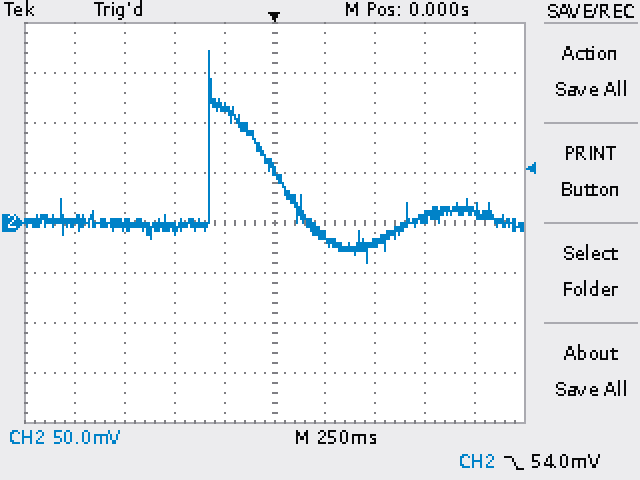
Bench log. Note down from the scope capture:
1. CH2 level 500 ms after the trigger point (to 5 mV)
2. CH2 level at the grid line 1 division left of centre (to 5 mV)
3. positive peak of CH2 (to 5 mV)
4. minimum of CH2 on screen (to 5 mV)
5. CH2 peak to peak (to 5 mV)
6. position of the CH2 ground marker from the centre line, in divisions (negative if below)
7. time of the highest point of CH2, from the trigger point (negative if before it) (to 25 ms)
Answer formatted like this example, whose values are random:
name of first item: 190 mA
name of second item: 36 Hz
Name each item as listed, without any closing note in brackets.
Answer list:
CH2 level 500 ms after the trigger point: -20 mV
CH2 level at the grid line 1 division left of centre: 115 mV
positive peak of CH2: 170 mV
minimum of CH2 on screen: -40 mV
CH2 peak to peak: 210 mV
position of the CH2 ground marker from the centre line, in divisions: 0.0 div
time of the highest point of CH2, from the trigger point (negative if before it): -325 ms
